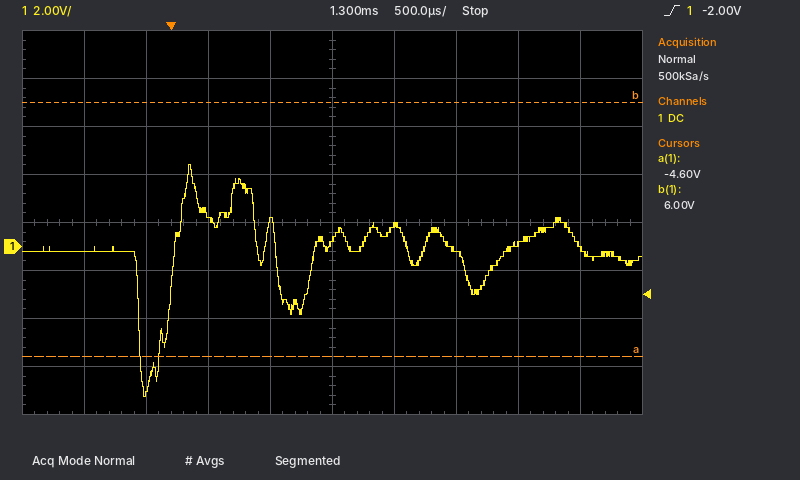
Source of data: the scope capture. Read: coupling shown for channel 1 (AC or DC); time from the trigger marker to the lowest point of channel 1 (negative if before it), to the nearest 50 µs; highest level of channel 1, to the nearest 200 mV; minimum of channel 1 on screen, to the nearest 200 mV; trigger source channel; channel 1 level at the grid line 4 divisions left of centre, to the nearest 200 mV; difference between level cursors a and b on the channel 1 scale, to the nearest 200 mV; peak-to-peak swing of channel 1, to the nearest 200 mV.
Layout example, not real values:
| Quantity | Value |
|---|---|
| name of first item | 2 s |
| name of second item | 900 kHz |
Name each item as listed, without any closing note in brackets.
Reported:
| Quantity | Value |
|---|---|
| coupling shown for channel 1 | DC |
| time from the trigger marker to the lowest point of channel 1 (negative if before it), to the nearest 50 µs | -200 µs |
| highest level of channel 1, to the nearest 200 mV | 3.4 V |
| minimum of channel 1 on screen, to the nearest 200 mV | -6.2 V |
| trigger source channel | channel 1 |
| channel 1 level at the grid line 4 divisions left of centre, to the nearest 200 mV | -200 mV |
| difference between level cursors a and b on the channel 1 scale, to the nearest 200 mV | 10.6 V |
| peak-to-peak swing of channel 1, to the nearest 200 mV | 9.6 V |
